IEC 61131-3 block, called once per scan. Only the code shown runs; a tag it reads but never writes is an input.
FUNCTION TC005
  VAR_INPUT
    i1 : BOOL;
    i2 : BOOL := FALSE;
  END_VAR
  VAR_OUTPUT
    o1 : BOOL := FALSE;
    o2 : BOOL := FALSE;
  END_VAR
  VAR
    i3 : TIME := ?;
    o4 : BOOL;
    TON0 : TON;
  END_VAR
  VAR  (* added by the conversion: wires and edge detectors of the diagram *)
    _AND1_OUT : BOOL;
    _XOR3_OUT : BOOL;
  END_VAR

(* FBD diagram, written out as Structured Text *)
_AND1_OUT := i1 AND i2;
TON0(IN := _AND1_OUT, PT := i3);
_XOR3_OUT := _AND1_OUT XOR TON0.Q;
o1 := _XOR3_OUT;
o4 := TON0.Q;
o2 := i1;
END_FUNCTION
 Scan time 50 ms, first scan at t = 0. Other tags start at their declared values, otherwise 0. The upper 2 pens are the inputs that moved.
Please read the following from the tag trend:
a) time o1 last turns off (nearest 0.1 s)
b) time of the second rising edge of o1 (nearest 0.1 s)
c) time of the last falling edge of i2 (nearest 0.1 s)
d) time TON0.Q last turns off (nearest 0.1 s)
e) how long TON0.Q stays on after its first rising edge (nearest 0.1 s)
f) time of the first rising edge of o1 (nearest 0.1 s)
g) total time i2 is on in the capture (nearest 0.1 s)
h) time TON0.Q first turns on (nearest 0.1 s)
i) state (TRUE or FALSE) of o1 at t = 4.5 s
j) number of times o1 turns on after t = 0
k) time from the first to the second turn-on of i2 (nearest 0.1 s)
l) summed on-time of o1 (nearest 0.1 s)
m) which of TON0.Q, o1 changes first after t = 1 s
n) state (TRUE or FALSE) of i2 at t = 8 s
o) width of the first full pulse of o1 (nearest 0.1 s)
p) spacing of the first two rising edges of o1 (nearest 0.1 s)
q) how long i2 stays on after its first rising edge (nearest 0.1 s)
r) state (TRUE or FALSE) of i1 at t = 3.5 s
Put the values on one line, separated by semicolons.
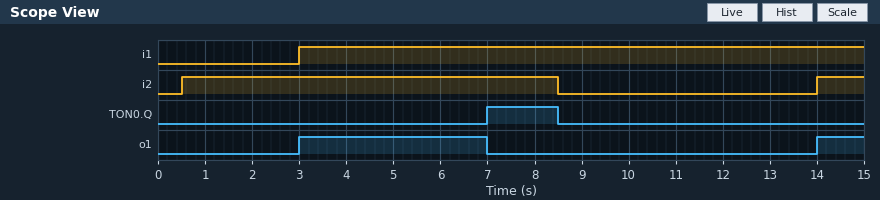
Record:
7.0 s; 14.0 s; 8.5 s; 8.5 s; 1.5 s; 3.0 s; 9.0 s; 7.0 s; TRUE; 2; 13.5 s; 5.0 s; o1; TRUE; 4.0 s; 11.0 s; 8.0 s; TRUE
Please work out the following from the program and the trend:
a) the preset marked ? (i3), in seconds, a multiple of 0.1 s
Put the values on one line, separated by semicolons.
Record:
4.0 s
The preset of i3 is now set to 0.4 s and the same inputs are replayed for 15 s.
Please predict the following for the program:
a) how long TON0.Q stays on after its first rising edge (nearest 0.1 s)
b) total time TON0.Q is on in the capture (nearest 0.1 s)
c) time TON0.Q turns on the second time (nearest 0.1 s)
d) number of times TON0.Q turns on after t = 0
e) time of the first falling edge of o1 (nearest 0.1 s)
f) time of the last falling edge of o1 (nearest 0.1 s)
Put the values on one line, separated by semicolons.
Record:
5.1 s; 5.7 s; 14.4 s; 2; 3.4 s; 14.4 s
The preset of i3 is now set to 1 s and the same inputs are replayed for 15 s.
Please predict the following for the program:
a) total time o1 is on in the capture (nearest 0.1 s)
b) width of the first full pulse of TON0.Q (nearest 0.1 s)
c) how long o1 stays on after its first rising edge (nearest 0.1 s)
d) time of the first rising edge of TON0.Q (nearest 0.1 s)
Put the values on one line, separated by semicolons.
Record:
2.0 s; 4.5 s; 1.0 s; 4.0 s
